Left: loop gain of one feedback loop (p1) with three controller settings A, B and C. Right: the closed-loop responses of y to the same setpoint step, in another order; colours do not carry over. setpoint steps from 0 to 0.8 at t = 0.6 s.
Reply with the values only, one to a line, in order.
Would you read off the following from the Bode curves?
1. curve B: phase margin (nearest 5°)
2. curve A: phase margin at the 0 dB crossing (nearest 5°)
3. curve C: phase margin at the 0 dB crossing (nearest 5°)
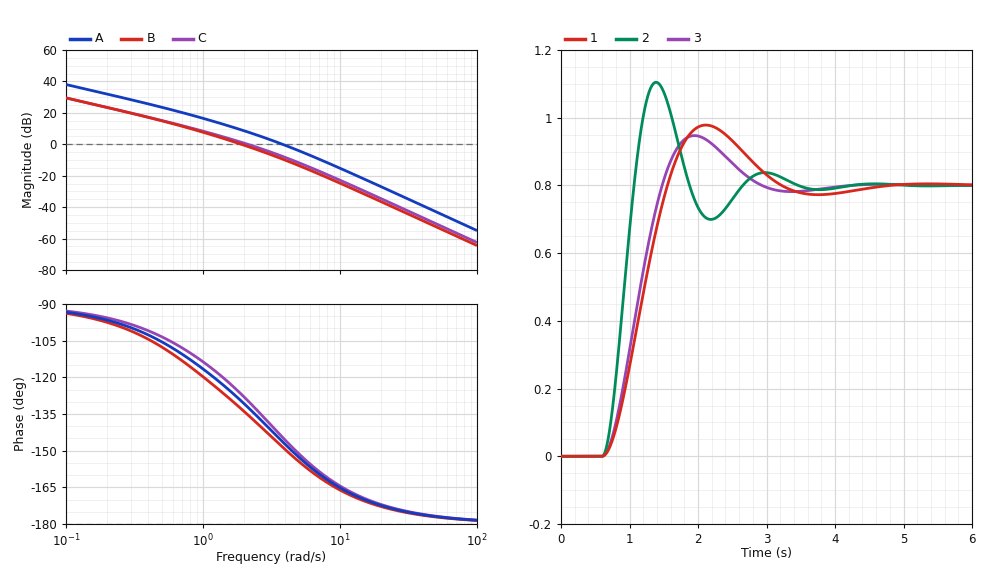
45°
35°
50°
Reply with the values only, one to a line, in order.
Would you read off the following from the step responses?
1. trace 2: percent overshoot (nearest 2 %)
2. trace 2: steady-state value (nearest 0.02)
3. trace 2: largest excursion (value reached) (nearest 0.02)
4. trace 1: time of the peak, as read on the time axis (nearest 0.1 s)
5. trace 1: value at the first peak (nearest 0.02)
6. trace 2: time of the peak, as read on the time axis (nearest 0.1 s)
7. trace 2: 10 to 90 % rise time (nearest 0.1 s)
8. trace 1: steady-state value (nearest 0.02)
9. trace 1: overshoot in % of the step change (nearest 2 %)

38 %
0.80
1.10
2.1 s
0.98
1.4 s
0.3 s
0.80
22 %
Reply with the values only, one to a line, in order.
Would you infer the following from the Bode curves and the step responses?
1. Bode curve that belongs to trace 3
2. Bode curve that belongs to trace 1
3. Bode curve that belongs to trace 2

C
B
A
